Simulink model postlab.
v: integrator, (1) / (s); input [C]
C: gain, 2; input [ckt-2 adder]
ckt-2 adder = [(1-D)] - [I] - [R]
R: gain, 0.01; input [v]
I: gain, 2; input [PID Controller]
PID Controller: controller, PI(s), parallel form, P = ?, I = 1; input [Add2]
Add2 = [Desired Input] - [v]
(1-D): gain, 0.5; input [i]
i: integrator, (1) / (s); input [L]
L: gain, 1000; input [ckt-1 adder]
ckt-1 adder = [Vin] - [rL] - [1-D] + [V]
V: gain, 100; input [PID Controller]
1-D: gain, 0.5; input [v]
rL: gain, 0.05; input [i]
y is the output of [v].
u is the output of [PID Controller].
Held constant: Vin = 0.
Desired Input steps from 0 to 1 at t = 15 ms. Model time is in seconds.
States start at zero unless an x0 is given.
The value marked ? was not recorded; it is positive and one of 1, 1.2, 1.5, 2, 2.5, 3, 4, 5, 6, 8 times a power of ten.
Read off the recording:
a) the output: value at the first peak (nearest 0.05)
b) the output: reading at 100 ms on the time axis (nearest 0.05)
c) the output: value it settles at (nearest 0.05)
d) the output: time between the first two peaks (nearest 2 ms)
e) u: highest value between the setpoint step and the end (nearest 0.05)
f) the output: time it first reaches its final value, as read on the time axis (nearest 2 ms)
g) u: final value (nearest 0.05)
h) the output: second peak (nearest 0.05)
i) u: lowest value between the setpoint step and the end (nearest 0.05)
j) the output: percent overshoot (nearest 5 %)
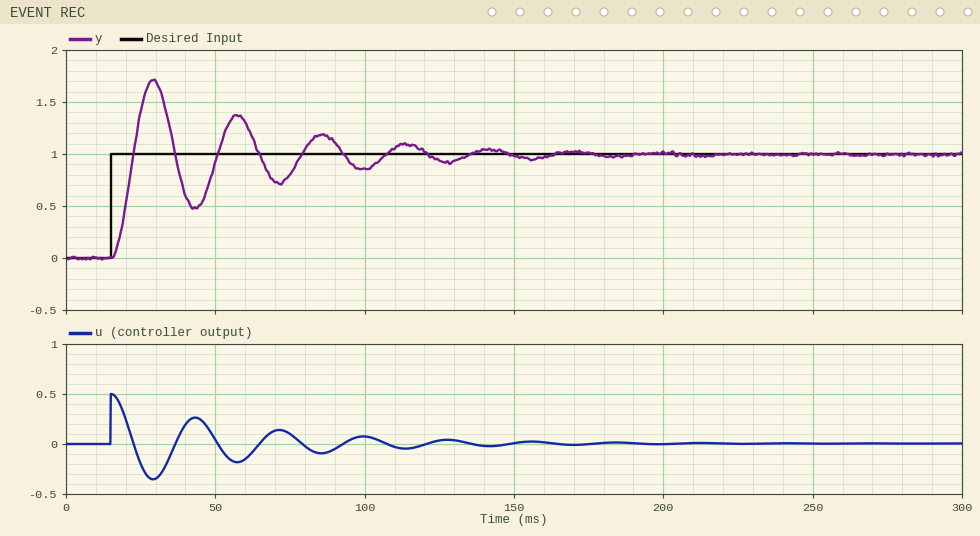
1.70
0.85
1.00
28 ms
0.50
22 ms
0.00
1.35
-0.35
70 %
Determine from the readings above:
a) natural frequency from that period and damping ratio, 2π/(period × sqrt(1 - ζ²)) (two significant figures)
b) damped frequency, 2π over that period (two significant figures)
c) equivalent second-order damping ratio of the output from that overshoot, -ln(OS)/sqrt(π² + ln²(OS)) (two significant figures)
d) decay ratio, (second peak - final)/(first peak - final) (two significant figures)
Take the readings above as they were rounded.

0.23 rad/ms
0.22 rad/ms
0.11
0.50
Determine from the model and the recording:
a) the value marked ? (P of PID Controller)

0.5
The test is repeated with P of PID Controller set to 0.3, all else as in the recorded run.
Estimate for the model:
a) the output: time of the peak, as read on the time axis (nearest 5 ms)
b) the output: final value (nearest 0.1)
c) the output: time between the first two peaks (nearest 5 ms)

35 ms
1.0
35 ms
